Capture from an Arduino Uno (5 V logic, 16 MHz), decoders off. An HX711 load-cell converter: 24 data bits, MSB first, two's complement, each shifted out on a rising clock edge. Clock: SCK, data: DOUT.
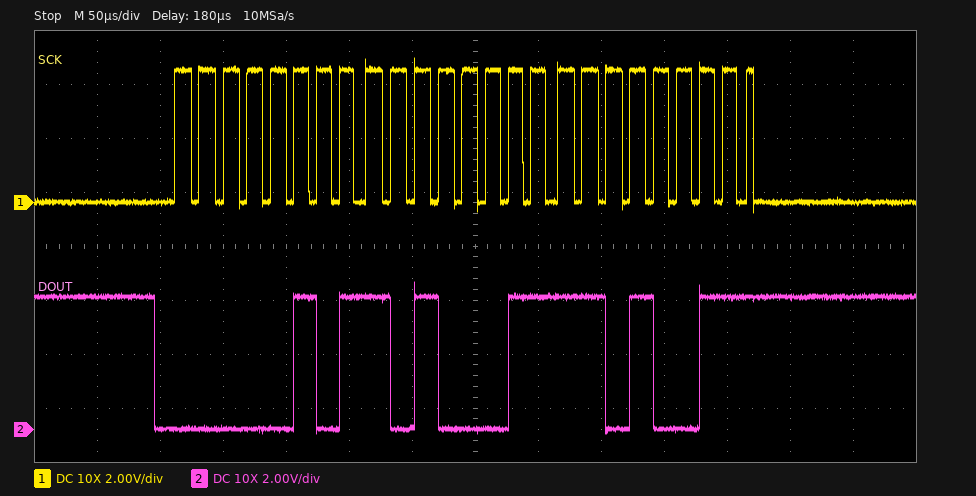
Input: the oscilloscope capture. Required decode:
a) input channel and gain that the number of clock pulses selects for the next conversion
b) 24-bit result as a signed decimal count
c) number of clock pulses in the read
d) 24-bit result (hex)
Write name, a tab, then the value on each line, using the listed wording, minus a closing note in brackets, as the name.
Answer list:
input channel and gain that the number of clock pulses selects for the next conversion	channel A, gain 128
24-bit result as a signed decimal count	369619
number of clock pulses in the read	25
24-bit result	0x05A3D3
